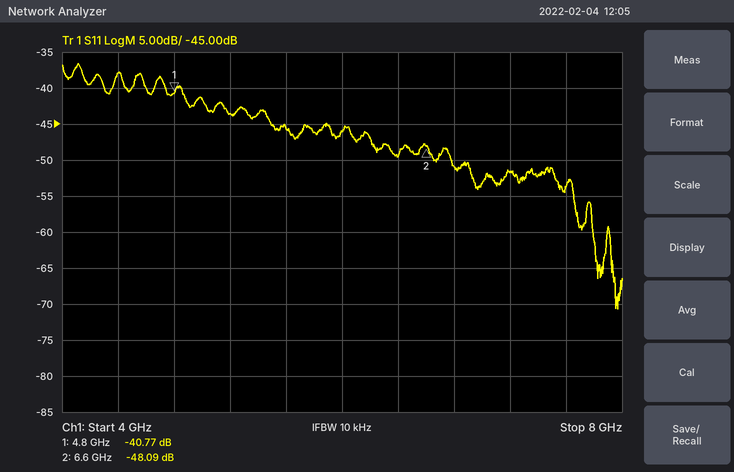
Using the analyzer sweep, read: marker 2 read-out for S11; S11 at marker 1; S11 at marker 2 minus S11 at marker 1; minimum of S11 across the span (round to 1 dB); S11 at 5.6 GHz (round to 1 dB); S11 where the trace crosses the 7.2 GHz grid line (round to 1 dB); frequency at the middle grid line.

-48.09 dB
-40.77 dB
-7.32 dB
-71 dB
-46 dB
-52 dB
6 GHz
